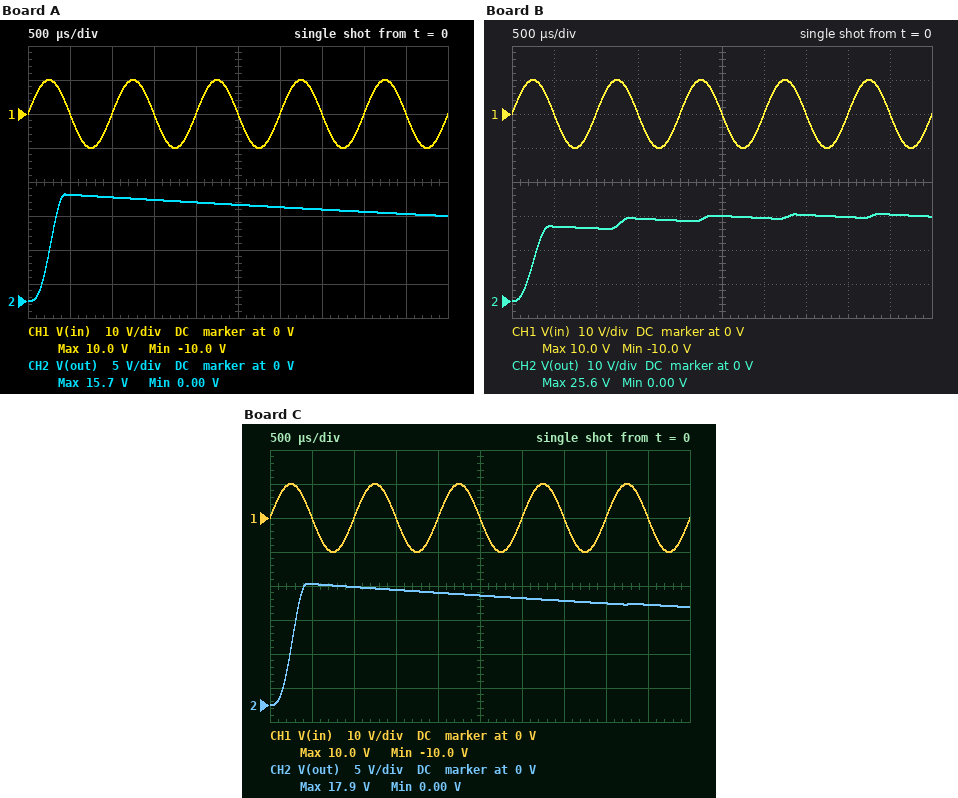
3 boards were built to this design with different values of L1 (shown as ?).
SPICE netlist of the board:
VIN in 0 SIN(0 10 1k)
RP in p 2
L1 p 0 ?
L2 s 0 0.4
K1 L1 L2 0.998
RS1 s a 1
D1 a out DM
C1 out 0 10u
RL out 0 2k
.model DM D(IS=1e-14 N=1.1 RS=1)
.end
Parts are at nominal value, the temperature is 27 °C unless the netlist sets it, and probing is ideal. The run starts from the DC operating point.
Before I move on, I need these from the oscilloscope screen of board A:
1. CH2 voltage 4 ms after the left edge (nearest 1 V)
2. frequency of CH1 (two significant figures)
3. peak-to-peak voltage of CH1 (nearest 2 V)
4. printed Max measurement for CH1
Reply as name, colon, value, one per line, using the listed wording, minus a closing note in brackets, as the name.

CH2 voltage 4 ms after the left edge: 13 V
frequency of CH1: 1.0 kHz
peak-to-peak voltage of CH1: 20 V
printed Max measurement for CH1: 10.0 V
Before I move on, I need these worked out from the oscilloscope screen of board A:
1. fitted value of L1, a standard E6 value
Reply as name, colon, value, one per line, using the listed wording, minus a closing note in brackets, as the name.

fitted value of L1, a standard E6 value: 220 mH
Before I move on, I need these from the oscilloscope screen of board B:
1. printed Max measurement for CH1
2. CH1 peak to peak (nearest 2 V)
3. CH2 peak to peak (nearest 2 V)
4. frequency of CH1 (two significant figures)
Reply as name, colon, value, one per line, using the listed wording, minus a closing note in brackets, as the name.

printed Max measurement for CH1: 10.0 V
CH1 peak to peak: 20 V
CH2 peak to peak: 26 V
frequency of CH1: 1.0 kHz
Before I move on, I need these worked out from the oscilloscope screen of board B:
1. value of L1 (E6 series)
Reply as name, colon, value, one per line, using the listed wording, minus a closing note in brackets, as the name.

value of L1: 47 mH
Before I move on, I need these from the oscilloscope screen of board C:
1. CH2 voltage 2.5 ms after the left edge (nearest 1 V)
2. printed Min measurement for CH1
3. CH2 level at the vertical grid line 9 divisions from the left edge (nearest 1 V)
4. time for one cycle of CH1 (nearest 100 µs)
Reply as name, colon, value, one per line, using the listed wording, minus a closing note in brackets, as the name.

CH2 voltage 2.5 ms after the left edge: 16 V
printed Min measurement for CH1: -10.0 V
CH2 level at the vertical grid line 9 divisions from the left edge: 15 V
time for one cycle of CH1: 1.0 ms
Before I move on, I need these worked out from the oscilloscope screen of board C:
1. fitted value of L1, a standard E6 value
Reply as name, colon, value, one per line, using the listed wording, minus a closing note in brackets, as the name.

fitted value of L1, a standard E6 value: 150 mH
